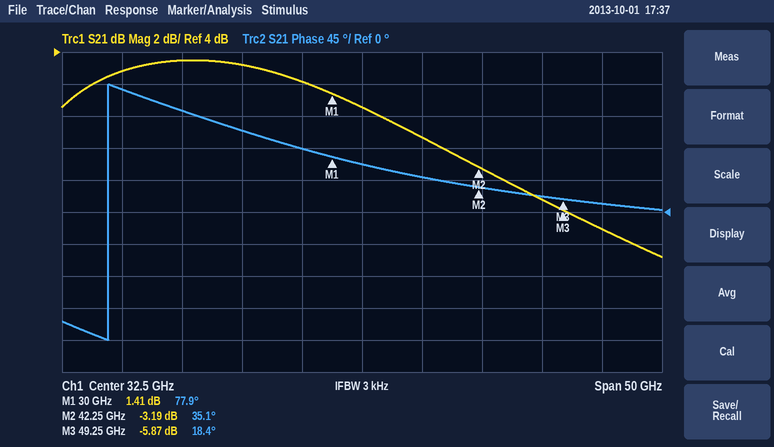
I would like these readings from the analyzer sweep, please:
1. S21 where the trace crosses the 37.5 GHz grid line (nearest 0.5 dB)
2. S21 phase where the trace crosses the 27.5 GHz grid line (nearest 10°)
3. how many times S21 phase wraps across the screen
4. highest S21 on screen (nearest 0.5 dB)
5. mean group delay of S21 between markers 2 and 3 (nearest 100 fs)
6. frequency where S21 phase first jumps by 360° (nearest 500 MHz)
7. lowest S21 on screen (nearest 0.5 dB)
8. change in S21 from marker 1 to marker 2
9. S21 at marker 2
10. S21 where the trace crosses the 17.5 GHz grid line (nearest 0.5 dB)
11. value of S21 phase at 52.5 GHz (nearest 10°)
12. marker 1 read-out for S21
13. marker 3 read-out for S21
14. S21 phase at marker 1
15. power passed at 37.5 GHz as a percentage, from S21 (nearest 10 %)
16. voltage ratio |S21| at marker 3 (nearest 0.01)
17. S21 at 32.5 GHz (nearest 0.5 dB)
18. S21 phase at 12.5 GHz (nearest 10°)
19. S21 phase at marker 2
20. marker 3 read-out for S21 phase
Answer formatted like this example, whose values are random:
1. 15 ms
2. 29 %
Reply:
1. -1.5 dB
2. 90°
3. 1
4. 3.5 dB
5. 6.6 ps
6. 11.5 GHz
7. -9.0 dB
8. -4.60 dB
9. -3.19 dB
10. 3.5 dB
11. 10°
12. 1.41 dB
13. -5.87 dB
14. 77.9°
15. 70 %
16. 0.51
17. 0.5 dB
18. 170°
19. 35.1°
20. 18.4°
